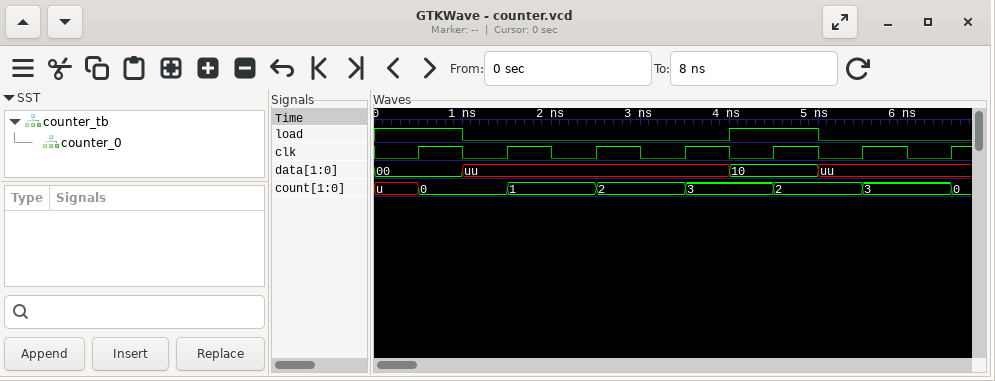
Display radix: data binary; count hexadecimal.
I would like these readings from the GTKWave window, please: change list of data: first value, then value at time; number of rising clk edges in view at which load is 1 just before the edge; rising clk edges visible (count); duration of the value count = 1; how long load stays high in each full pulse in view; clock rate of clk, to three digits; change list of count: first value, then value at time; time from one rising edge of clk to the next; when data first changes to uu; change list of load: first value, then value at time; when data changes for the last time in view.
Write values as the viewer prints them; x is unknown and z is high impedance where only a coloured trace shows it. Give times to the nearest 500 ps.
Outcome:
00, uu at 1000 ps, 10 at 4000 ps, uu at 5000 ps
2
7
1000 ps
1000 ps
1.00 GHz
u, 0 at 500 ps, 1 at 1500 ps, 2 at 2500 ps, 3 at 3500 ps, 2 at 4500 ps, 3 at 5500 ps, 0 at 6500 ps
1000 ps
1000 ps
1, 0 at 1000 ps, 1 at 4000 ps, 0 at 5000 ps
5000 ps
